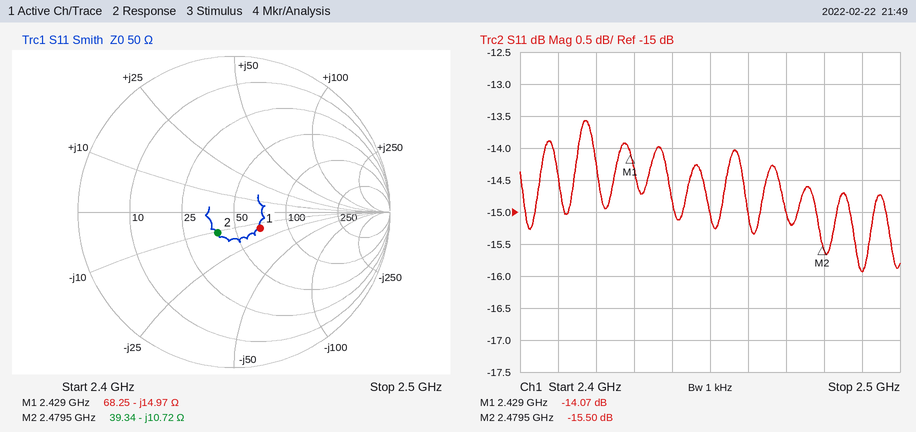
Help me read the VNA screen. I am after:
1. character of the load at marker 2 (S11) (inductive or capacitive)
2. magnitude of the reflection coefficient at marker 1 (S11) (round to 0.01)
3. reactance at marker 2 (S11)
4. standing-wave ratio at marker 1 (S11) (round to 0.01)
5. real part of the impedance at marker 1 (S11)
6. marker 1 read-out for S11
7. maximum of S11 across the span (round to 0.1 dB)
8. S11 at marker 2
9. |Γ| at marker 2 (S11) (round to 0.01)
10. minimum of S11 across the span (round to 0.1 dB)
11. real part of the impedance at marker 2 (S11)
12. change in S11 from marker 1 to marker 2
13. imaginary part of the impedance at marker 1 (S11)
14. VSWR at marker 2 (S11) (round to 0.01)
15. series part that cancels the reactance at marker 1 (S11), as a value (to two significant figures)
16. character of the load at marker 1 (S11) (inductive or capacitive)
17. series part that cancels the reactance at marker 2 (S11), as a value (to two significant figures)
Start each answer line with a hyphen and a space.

- capacitive
- 0.20
- -10.72 Ω
- 1.49
- 68.25 Ω
- -14.07 dB
- -13.6 dB
- -15.50 dB
- 0.17
- -15.9 dB
- 39.34 Ω
- -1.43 dB
- -14.97 Ω
- 1.40
- 980 pH
- capacitive
- 690 pH
